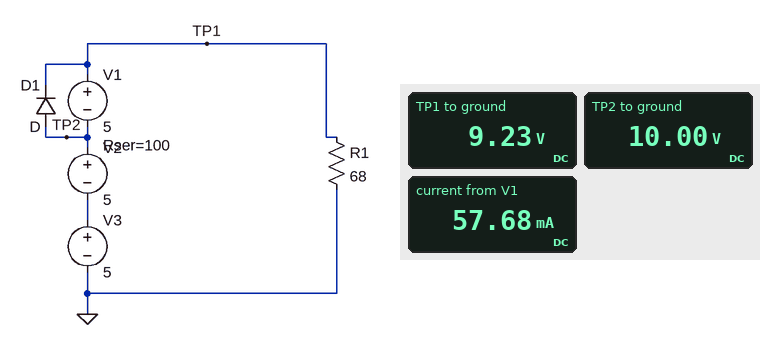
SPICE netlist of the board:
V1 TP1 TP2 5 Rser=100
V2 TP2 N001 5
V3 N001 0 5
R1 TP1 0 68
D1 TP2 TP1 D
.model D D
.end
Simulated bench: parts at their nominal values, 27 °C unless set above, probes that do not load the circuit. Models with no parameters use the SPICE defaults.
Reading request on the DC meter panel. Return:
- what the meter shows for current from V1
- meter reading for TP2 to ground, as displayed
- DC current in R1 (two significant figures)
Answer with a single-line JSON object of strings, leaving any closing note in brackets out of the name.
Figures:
{"what the meter shows for current from V1": "57.68 mA", "meter reading for TP2 to ground, as displayed": "10.00 V", "DC current in R1": "140 mA"}
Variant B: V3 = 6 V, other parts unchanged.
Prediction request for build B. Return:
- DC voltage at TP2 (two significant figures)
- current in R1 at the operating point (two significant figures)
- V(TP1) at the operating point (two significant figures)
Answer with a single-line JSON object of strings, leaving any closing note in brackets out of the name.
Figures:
{"DC voltage at TP2": "11 V", "current in R1 at the operating point": "150 mA", "V(TP1) at the operating point": "10 V"}
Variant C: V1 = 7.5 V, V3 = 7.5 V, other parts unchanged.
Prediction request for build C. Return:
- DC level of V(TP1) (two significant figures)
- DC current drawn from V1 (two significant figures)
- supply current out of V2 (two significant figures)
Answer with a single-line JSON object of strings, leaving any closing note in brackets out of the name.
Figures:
{"DC level of V(TP1)": "12 V", "DC current drawn from V1": "83 mA", "supply current out of V2": "170 mA"}
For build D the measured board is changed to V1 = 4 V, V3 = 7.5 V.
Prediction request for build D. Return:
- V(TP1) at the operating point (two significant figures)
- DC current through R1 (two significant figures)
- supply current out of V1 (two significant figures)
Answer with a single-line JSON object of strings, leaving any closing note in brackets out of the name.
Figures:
{"V(TP1) at the operating point": "12 V", "DC current through R1": "170 mA", "supply current out of V1": "48 mA"}
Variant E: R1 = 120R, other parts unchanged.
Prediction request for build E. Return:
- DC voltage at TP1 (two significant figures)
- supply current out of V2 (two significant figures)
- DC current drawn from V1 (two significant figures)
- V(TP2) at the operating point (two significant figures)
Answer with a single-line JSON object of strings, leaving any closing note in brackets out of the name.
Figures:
{"DC voltage at TP1": "9.3 V", "supply current out of V2": "77 mA", "DC current drawn from V1": "57 mA", "V(TP2) at the operating point": "10 V"}
